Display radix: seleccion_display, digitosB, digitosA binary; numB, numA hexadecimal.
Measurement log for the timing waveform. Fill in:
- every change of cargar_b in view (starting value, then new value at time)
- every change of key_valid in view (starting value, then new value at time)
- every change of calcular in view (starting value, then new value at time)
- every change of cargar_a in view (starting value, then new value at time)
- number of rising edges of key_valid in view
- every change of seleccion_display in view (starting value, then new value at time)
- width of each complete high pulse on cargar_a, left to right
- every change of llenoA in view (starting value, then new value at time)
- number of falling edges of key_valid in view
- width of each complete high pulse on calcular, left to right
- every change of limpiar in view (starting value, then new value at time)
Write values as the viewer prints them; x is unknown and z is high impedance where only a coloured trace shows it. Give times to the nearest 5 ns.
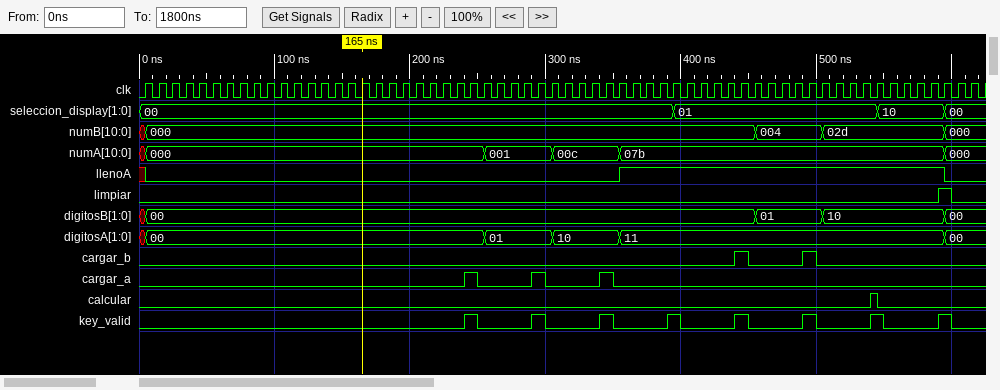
0, 1 at 440 ns, 0 at 450 ns, 1 at 490 ns, 0 at 500 ns
0, 1 at 240 ns, 0 at 250 ns, 1 at 290 ns, 0 at 300 ns, 1 at 340 ns, 0 at 350 ns, 1 at 390 ns, 0 at 400 ns, 1 at 440 ns, 0 at 450 ns, 1 at 490 ns, 0 at 500 ns, 1 at 540 ns, 0 at 550 ns, 1 at 590 ns, 0 at 600 ns
0, 1 at 540 ns, 0 at 545 ns
0, 1 at 240 ns, 0 at 250 ns, 1 at 290 ns, 0 at 300 ns, 1 at 340 ns, 0 at 350 ns
8
00, 01 at 395 ns, 10 at 545 ns, 00 at 595 ns
10 ns, 10 ns, 10 ns
x, 0 at 5 ns, 1 at 355 ns, 0 at 595 ns
8
5 ns
0, 1 at 590 ns, 0 at 600 ns
